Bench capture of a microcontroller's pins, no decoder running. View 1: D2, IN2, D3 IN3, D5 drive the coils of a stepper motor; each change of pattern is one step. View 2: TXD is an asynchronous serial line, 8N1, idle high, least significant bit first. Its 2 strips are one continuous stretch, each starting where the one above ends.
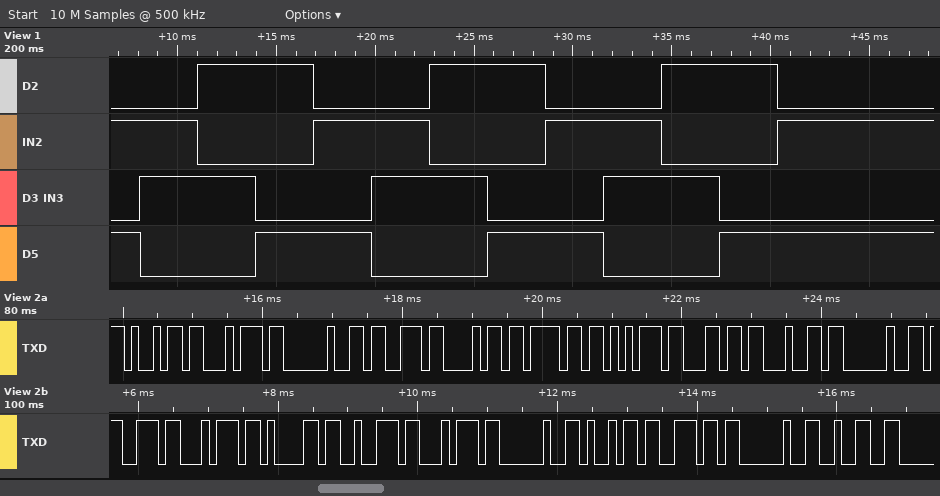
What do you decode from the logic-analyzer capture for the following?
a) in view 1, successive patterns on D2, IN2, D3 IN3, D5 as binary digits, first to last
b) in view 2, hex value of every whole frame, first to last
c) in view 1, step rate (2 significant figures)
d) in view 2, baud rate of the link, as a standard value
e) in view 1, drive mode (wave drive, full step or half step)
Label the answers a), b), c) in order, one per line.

a) 0101 0110 1010 1001 0101 0110 1010 1001 0101 0110 1010 1001 0101
b) 69 74 20 73 68 6F 75 6C 64 20 73 74 61 72 74 20 69 6E 20 32
c) 340 steps/s
d) 9600 baud
e) full step
